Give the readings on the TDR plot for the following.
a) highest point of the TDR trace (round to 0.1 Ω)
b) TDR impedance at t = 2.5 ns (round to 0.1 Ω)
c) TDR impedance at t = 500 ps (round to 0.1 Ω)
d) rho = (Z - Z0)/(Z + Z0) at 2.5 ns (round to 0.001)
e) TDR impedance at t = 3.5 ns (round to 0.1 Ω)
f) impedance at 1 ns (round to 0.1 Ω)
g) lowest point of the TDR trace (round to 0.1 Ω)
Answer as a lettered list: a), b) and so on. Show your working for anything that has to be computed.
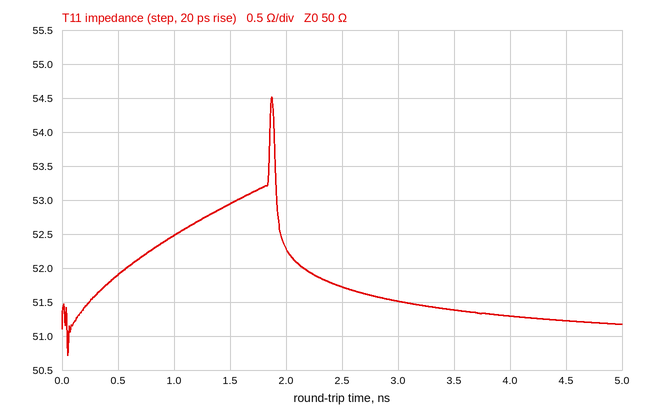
a) 54.5 Ω
b) 51.7 Ω
c) 51.9 Ω
d) (51.7 − 50)/(51.7 + 50) ≈ +0.017
e) 51.4 Ω
f) 52.5 Ω
g) 50.7 Ω
